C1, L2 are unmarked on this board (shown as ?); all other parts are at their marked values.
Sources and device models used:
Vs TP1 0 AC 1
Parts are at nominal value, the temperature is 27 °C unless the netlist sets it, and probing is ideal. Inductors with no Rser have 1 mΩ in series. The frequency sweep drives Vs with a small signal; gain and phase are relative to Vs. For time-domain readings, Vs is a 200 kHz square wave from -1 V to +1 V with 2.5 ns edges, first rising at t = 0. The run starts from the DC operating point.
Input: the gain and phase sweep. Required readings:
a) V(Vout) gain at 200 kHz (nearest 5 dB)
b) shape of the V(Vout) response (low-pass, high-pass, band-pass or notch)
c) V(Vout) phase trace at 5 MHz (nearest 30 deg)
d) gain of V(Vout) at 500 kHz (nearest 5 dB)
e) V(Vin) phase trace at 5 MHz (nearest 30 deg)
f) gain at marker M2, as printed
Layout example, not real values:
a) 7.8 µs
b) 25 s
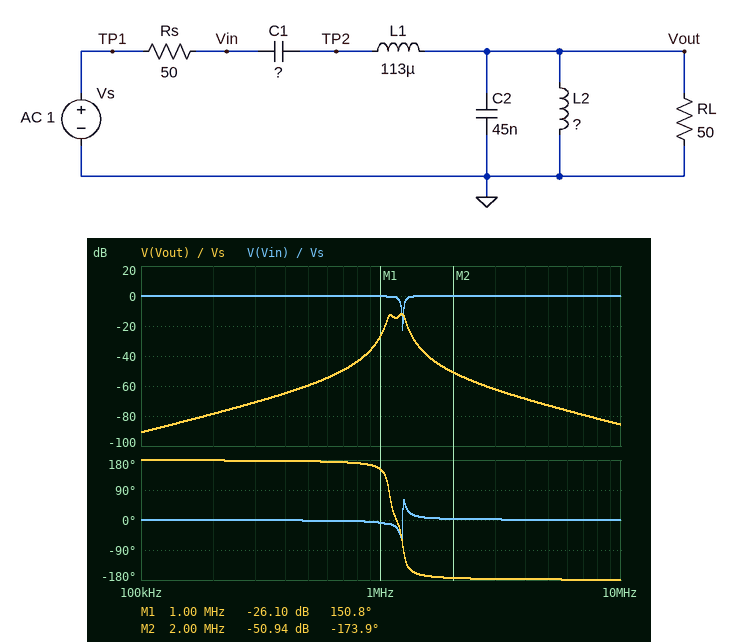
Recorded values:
a) -80 dB
b) band-pass
c) -180 deg
d) -60 dB
e) 0 deg
f) -50.94 dB
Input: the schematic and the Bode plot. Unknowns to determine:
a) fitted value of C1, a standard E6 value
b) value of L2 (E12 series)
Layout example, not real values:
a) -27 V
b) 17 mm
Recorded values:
a) 150 pF
b) 470 nH
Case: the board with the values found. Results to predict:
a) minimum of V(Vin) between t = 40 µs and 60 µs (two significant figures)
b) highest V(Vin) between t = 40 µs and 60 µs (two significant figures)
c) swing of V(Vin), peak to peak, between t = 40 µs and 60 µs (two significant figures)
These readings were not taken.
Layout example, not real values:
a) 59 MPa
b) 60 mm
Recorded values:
a) -1.1 V
b) 1.1 V
c) 2.1 V
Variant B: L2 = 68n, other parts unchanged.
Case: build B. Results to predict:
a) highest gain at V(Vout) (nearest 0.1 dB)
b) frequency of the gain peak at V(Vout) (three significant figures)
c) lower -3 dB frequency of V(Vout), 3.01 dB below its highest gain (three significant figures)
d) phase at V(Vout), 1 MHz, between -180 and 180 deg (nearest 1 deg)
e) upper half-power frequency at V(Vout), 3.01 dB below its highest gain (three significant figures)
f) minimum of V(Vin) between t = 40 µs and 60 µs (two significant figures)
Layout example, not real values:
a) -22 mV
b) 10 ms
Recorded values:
a) -30.8 dB
b) 2.88 MHz
c) 2.84 MHz
d) 171 deg
e) 2.91 MHz
f) -1.1 V
